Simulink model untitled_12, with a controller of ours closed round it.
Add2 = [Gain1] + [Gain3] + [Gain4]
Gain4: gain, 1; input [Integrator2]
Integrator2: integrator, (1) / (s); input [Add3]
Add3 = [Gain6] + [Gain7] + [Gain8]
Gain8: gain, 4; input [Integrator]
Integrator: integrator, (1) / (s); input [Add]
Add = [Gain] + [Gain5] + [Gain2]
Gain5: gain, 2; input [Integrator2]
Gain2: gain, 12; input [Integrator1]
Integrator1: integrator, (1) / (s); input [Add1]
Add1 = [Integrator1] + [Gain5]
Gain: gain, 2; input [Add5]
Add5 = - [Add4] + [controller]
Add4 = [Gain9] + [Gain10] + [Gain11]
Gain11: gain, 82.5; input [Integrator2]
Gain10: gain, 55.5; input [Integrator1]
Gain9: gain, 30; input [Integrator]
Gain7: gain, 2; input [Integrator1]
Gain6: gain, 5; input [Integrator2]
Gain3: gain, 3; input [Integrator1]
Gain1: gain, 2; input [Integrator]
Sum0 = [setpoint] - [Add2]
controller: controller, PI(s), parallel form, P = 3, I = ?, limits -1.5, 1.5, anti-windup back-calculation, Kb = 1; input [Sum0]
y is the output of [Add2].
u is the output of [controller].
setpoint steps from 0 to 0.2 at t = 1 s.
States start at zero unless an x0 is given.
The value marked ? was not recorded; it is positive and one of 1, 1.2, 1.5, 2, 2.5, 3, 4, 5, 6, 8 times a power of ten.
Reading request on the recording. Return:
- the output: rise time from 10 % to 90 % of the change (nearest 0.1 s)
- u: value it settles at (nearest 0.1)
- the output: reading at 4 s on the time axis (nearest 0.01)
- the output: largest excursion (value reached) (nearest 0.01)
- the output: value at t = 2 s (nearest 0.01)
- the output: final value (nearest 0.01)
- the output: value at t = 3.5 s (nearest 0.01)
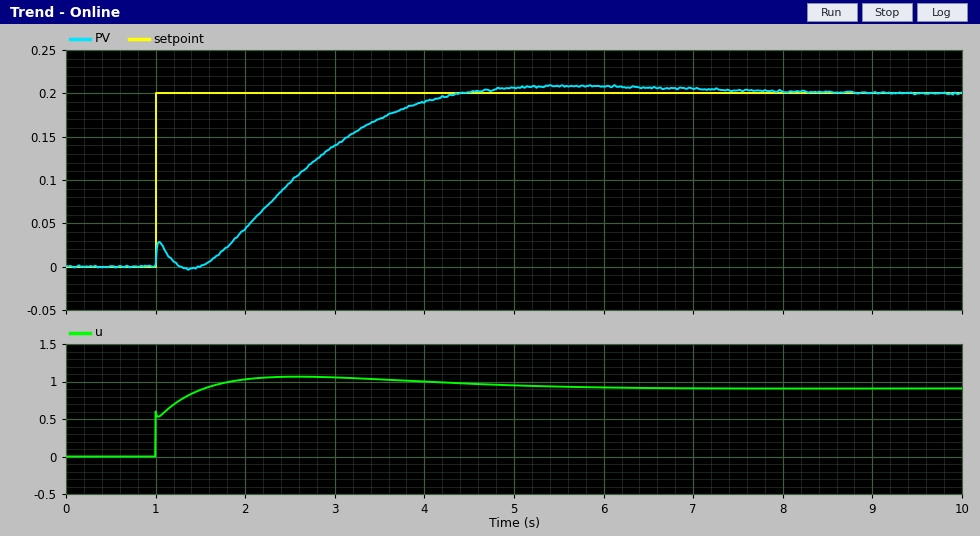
2.7 s
0.9
0.19
0.21
0.04
0.20
0.17
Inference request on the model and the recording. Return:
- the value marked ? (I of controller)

3
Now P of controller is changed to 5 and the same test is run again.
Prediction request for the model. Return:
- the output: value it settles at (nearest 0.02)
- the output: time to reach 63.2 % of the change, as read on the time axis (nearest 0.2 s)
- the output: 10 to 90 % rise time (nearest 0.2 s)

0.20
2.4 s
2.2 s
